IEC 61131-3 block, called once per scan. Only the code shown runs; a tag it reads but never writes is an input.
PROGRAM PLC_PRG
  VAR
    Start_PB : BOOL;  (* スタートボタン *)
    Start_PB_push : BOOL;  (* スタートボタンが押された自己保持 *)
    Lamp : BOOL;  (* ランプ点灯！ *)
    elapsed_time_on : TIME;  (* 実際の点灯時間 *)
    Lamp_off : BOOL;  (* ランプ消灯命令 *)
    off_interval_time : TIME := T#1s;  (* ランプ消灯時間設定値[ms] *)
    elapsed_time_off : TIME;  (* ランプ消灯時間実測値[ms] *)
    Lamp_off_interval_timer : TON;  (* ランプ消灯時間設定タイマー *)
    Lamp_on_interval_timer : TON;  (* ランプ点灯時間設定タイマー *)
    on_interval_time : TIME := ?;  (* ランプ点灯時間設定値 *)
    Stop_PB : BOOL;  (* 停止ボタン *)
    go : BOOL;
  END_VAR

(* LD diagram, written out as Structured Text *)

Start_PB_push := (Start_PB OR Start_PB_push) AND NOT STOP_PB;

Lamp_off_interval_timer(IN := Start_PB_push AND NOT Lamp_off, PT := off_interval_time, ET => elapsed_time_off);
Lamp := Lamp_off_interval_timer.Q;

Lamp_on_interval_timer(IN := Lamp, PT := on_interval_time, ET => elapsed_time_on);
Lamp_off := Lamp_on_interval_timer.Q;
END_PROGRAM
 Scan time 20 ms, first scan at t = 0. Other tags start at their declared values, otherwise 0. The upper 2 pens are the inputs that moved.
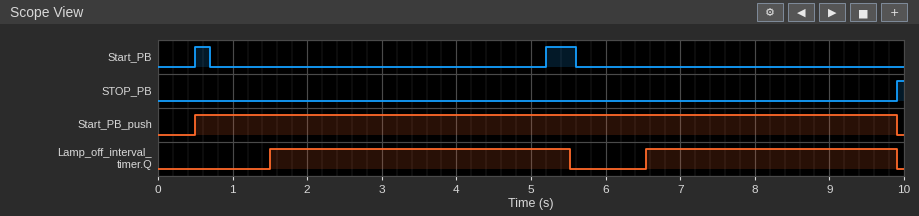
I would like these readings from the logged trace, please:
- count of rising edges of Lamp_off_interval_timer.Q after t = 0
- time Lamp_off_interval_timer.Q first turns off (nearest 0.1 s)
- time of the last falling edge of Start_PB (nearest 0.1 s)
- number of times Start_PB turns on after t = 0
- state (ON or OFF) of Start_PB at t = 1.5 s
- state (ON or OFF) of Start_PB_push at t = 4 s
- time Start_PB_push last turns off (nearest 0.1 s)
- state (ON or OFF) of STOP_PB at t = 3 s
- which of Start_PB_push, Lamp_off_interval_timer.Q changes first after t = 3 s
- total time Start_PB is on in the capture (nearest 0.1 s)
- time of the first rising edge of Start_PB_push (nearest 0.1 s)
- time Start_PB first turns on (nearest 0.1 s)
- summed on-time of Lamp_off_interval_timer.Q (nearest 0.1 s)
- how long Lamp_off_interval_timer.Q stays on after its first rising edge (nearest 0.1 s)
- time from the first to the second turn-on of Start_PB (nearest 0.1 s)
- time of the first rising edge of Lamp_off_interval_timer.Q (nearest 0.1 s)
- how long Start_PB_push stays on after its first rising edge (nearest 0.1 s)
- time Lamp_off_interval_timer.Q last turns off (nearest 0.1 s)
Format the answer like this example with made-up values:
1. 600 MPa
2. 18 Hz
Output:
1. 2
2. 5.5 s
3. 5.6 s
4. 2
5. OFF
6. ON
7. 9.9 s
8. OFF
9. Lamp_off_interval_timer.Q
10. 0.6 s
11. 0.5 s
12. 0.5 s
13. 7.4 s
14. 4.0 s
15. 4.7 s
16. 1.5 s
17. 9.4 s
18. 9.9 s
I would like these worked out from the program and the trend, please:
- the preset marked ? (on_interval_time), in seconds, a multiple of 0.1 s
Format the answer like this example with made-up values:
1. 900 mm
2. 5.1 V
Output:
1. 4.0 s
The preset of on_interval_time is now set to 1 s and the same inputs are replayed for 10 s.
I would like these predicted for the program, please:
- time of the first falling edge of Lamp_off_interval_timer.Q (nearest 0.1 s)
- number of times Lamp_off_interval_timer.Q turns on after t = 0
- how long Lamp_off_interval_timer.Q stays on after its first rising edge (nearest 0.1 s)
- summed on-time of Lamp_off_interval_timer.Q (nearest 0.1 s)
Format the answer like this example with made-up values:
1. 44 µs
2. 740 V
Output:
1. 2.5 s
2. 5
3. 1.0 s
4. 4.3 s
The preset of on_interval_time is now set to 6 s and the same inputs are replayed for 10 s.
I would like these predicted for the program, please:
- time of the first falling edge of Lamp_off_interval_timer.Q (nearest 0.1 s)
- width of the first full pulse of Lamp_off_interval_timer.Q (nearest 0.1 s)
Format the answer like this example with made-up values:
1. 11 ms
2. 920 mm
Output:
1. 7.5 s
2. 6.0 s
